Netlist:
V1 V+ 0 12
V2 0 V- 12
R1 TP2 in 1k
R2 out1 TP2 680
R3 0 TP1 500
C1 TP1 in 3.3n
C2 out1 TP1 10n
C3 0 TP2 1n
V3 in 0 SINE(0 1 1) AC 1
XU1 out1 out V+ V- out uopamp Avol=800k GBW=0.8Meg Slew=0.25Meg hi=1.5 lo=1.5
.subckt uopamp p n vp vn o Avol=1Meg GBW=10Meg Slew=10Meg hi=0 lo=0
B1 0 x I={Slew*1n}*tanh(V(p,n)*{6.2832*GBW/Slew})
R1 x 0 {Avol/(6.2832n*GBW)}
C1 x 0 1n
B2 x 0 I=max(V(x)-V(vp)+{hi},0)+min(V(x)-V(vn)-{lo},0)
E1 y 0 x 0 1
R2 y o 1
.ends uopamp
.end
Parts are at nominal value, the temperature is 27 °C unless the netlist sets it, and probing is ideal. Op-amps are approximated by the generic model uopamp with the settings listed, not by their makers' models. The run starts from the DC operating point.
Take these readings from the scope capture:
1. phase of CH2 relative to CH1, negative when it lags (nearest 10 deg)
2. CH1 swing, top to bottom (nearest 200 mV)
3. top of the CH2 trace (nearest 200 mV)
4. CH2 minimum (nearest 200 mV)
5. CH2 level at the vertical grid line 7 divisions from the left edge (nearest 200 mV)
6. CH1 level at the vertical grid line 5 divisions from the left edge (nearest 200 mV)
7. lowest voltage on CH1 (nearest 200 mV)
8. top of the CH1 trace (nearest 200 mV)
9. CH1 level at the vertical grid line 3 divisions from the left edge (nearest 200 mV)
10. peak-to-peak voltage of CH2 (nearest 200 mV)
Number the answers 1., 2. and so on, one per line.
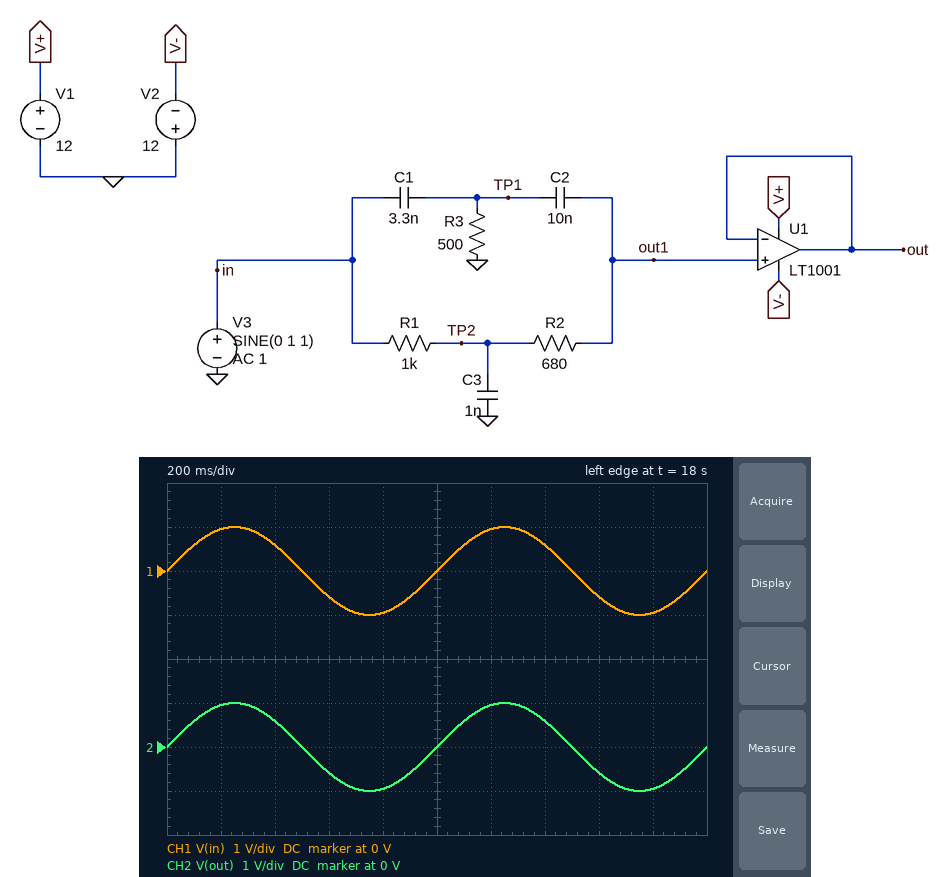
1. 0 deg
2. 2.0 V
3. 1.0 V
4. -1.0 V
5. 600 mV
6. 0 V
7. -1.0 V
8. 1.0 V
9. -600 mV
10. 2.0 V
